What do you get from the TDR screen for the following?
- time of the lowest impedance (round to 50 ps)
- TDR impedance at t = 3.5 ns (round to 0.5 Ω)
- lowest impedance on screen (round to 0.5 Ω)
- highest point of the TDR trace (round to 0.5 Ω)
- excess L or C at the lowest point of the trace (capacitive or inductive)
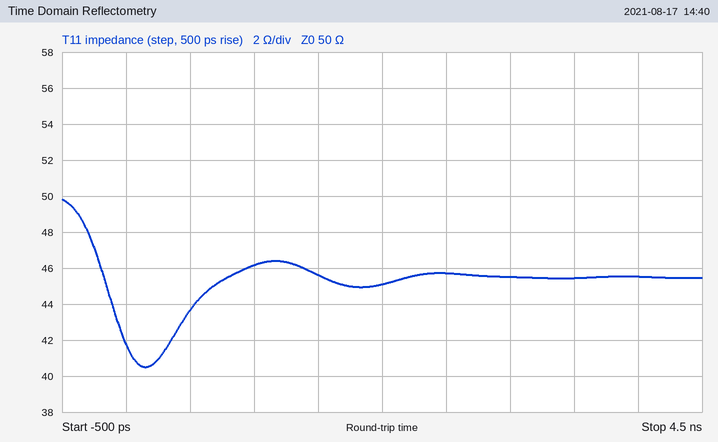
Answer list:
150 ps
45.5 Ω
40.5 Ω
50.0 Ω
capacitive
